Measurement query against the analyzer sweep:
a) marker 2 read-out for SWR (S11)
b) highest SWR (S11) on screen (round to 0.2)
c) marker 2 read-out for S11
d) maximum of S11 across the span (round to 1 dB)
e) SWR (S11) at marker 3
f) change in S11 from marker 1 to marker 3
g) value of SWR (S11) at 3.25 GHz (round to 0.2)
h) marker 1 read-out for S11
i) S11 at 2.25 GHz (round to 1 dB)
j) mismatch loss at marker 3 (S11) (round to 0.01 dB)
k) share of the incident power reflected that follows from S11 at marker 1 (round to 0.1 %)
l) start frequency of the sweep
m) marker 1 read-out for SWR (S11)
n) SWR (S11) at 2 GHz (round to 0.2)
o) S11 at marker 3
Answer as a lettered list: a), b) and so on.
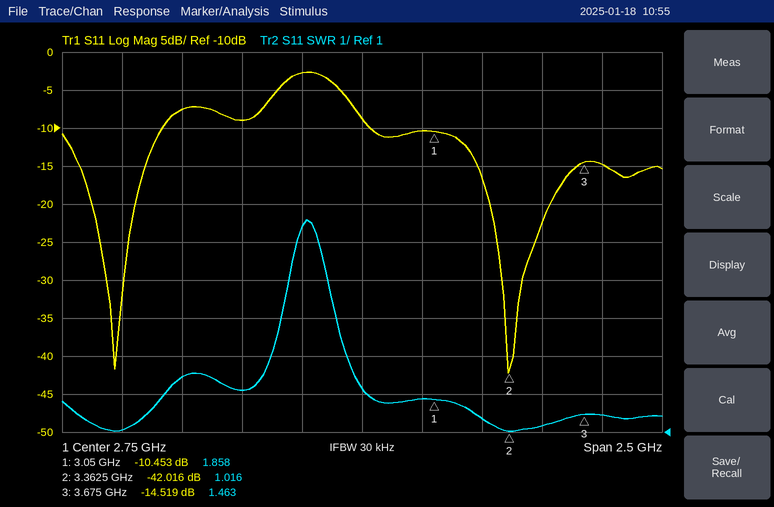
a) 1.016
b) 6.6
c) -42.016 dB
d) -3 dB
e) 1.463
f) -4.066 dB
g) 1.4
h) -10.453 dB
i) -9 dB
j) 0.16 dB
k) 9.0 %
l) 1.5 GHz
m) 1.858
n) 2.4
o) -14.519 dB
